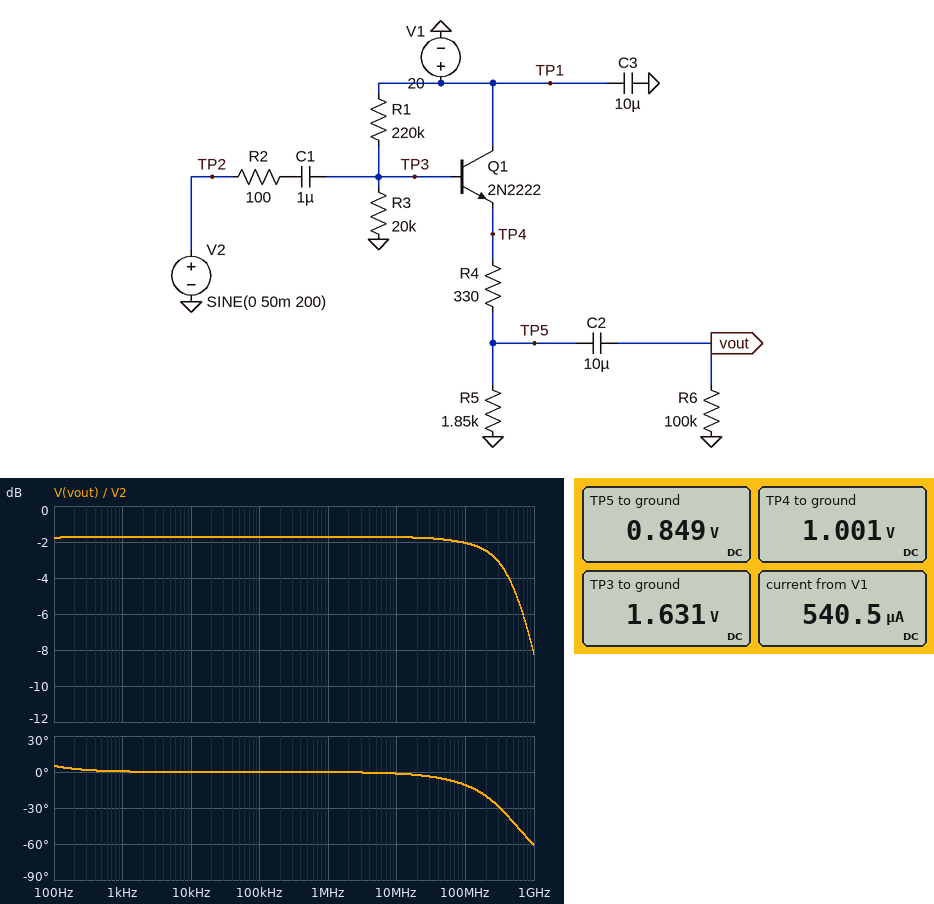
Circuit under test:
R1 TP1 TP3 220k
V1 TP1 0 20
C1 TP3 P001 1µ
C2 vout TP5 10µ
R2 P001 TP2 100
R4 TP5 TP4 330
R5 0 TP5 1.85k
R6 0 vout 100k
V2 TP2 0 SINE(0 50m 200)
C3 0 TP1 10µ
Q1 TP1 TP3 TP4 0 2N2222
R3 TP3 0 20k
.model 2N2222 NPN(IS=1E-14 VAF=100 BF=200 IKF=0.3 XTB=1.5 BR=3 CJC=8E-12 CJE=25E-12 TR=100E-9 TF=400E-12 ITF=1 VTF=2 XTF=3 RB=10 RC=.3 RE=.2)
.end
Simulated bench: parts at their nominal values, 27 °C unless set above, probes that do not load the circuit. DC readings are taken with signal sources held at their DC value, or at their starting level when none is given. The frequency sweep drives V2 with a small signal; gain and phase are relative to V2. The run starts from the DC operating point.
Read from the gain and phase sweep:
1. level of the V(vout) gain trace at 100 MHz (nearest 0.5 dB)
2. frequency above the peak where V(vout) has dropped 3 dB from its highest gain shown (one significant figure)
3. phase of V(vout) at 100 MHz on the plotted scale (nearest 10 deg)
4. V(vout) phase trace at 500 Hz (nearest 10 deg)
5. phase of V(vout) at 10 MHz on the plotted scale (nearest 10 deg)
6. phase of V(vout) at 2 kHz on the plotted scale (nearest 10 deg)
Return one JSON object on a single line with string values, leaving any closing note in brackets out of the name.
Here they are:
{"level of the V(vout) gain trace at 100 MHz": "-2.0 dB", "frequency above the peak where V(vout) has dropped 3 dB from its highest gain shown": "500 MHz", "phase of V(vout) at 100 MHz on the plotted scale": "-10 deg", "V(vout) phase trace at 500 Hz": "0 deg", "phase of V(vout) at 10 MHz on the plotted scale": "0 deg", "phase of V(vout) at 2 kHz on the plotted scale": "0 deg"}
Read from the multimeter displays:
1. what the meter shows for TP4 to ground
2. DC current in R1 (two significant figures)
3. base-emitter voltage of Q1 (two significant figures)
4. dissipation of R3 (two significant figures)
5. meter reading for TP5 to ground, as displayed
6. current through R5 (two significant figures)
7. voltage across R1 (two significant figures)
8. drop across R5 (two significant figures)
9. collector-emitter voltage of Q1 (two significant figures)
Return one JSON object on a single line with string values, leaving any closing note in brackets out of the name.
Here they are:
{"what the meter shows for TP4 to ground": "1.001 V", "DC current in R1": "83 µA", "base-emitter voltage of Q1": "630 mV", "dissipation of R3": "130 µW", "meter reading for TP5 to ground, as displayed": "0.849 V", "current through R5": "460 µA", "voltage across R1": "18 V", "drop across R5": "850 mV", "collector-emitter voltage of Q1": "19 V"}
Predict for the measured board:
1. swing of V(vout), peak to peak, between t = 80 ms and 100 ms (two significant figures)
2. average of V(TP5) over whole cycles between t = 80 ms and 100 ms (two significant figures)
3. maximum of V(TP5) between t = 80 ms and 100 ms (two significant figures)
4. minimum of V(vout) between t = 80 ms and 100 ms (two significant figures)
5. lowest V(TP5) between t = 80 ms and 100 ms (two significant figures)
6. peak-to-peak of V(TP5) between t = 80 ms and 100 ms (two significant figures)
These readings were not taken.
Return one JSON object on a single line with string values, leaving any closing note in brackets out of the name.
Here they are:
{"swing of V(vout), peak to peak, between t = 80 ms and 100 ms": "82 mV", "average of V(TP5) over whole cycles between t = 80 ms and 100 ms": "850 mV", "maximum of V(TP5) between t = 80 ms and 100 ms": "890 mV", "minimum of V(vout) between t = 80 ms and 100 ms": "-41 mV", "lowest V(TP5) between t = 80 ms and 100 ms": "810 mV", "peak-to-peak of V(TP5) between t = 80 ms and 100 ms": "82 mV"}
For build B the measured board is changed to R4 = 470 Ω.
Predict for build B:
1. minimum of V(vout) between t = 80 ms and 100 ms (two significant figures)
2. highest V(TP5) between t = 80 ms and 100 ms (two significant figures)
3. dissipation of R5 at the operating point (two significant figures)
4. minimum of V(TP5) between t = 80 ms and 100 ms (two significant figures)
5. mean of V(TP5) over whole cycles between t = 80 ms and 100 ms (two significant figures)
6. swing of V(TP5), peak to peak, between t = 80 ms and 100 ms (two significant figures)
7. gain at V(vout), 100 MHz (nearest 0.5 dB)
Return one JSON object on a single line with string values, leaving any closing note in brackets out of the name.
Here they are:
{"minimum of V(vout) between t = 80 ms and 100 ms": "-38 mV", "highest V(TP5) between t = 80 ms and 100 ms": "840 mV", "dissipation of R5 at the operating point": "350 µW", "minimum of V(TP5) between t = 80 ms and 100 ms": "760 mV", "mean of V(TP5) over whole cycles between t = 80 ms and 100 ms": "800 mV", "swing of V(TP5), peak to peak, between t = 80 ms and 100 ms": "77 mV", "gain at V(vout), 100 MHz": "-2.5 dB"}
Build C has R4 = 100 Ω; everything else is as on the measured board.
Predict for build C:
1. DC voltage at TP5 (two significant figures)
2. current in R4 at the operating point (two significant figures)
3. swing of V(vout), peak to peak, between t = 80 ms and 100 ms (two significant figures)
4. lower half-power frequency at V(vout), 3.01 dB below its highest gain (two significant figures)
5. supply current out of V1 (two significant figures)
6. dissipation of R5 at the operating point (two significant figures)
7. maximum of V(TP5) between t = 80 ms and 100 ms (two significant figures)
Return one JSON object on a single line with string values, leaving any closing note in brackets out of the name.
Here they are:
{"DC voltage at TP5": "940 mV", "current in R4 at the operating point": "510 µA", "swing of V(vout), peak to peak, between t = 80 ms and 100 ms": "92 mV", "lower half-power frequency at V(vout), 3.01 dB below its highest gain": "9.0 Hz", "supply current out of V1": "590 µA", "dissipation of R5 at the operating point": "480 µW", "maximum of V(TP5) between t = 80 ms and 100 ms": "990 mV"}
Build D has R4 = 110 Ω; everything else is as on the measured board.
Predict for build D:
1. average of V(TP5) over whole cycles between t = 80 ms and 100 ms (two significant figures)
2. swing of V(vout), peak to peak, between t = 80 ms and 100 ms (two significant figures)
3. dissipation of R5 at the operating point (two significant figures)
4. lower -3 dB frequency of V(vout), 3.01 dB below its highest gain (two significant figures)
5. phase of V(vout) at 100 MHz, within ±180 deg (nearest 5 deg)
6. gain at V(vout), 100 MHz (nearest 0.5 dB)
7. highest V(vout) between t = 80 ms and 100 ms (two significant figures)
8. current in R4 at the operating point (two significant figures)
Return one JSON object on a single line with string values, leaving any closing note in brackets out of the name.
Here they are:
{"average of V(TP5) over whole cycles between t = 80 ms and 100 ms": "940 mV", "swing of V(vout), peak to peak, between t = 80 ms and 100 ms": "91 mV", "dissipation of R5 at the operating point": "480 µW", "lower -3 dB frequency of V(vout), 3.01 dB below its highest gain": "9.0 Hz", "phase of V(vout) at 100 MHz, within ±180 deg": "-10 deg", "gain at V(vout), 100 MHz": "-1.0 dB", "highest V(vout) between t = 80 ms and 100 ms": "46 mV", "current in R4 at the operating point": "510 µA"}
